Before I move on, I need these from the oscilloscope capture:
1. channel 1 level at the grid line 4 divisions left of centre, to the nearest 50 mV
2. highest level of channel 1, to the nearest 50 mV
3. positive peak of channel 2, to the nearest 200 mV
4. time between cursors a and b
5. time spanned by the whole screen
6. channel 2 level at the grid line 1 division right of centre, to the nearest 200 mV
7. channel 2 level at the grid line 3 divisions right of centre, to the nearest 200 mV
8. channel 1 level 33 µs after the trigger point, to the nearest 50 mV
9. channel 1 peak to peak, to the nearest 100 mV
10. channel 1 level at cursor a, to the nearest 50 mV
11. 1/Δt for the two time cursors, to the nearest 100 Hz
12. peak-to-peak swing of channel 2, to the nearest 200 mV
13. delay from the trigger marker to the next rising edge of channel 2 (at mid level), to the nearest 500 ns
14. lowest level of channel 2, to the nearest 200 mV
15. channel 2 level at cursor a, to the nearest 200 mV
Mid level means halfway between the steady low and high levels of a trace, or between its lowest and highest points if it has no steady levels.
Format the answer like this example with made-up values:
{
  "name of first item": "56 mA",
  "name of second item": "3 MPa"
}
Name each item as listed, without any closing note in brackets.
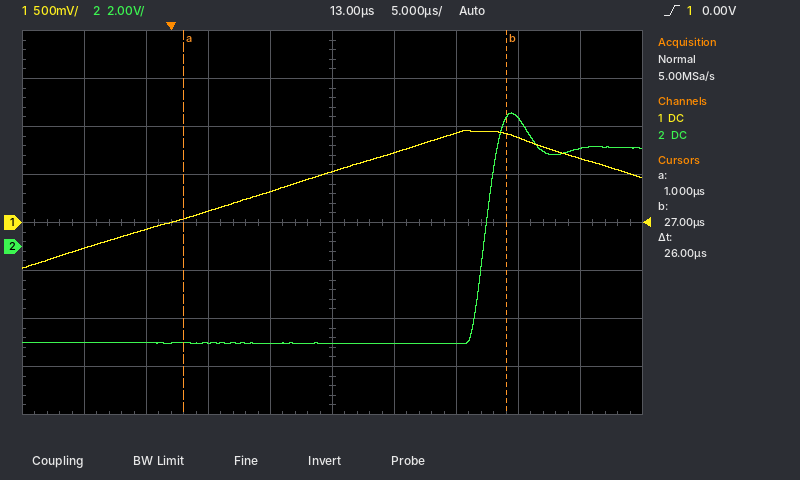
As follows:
{
  "channel 1 level at the grid line 4 divisions left of centre, to the nearest 50 mV": "-250 mV",
  "highest level of channel 1, to the nearest 50 mV": "950 mV",
  "positive peak of channel 2, to the nearest 200 mV": "5.6 V",
  "time between cursors a and b": "26 µs",
  "time spanned by the whole screen": "50 µs",
  "channel 2 level at the grid line 1 division right of centre, to the nearest 200 mV": "-4.0 V",
  "channel 2 level at the grid line 3 divisions right of centre, to the nearest 200 mV": "5.4 V",
  "channel 1 level 33 µs after the trigger point, to the nearest 50 mV": "650 mV",
  "channel 1 peak to peak, to the nearest 100 mV": "1.40 V",
  "channel 1 level at cursor a, to the nearest 50 mV": "50 mV",
  "1/Δt for the two time cursors, to the nearest 100 Hz": "38.5 kHz",
  "peak-to-peak swing of channel 2, to the nearest 200 mV": "9.6 V",
  "delay from the trigger marker to the next rising edge of channel 2 (at mid level), to the nearest 500 ns": "25.5 µs",
  "lowest level of channel 2, to the nearest 200 mV": "-4.0 V",
  "channel 2 level at cursor a, to the nearest 200 mV": "-4.0 V"
}
